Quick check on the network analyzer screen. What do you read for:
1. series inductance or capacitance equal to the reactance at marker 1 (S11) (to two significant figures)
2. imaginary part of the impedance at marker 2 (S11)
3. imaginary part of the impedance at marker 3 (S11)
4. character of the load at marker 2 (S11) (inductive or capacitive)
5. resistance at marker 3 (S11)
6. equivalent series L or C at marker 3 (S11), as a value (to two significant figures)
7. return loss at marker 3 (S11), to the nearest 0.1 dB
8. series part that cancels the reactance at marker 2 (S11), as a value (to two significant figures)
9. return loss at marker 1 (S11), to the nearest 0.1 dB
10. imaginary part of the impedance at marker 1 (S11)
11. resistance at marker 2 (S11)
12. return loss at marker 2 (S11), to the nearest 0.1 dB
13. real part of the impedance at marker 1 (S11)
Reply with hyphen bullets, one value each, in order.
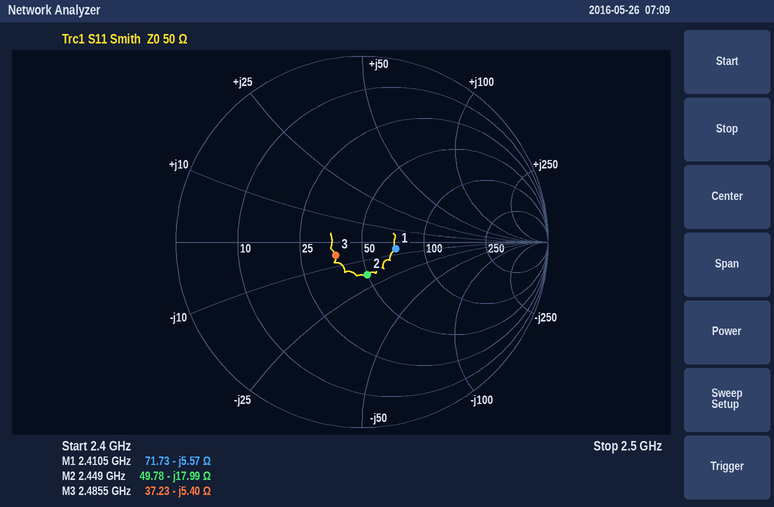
- 12 pF
- -17.99 Ω
- -5.40 Ω
- capacitive
- 37.23 Ω
- 12 pF
- 16.0 dB
- 1.2 nH
- 14.7 dB
- -5.57 Ω
- 49.78 Ω
- 15.0 dB
- 71.73 Ω
